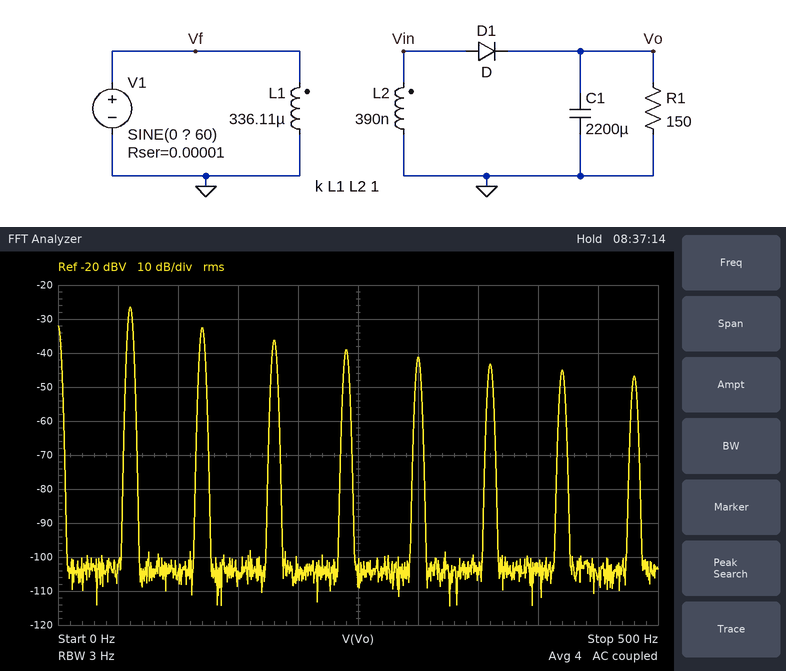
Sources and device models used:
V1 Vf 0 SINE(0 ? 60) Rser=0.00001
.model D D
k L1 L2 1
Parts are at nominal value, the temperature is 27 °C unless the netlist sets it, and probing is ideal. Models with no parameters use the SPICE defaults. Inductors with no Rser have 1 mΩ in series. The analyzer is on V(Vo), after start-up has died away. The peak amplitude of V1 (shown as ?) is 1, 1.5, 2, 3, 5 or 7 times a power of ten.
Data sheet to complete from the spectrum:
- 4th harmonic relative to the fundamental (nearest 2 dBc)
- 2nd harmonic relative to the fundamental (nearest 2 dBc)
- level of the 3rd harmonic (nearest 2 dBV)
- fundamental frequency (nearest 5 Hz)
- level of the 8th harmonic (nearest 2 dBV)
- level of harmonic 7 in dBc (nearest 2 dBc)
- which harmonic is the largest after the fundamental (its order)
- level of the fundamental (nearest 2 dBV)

-12 dBc
-6 dBc
-36 dBV
60 Hz
-46 dBV
-18 dBc
2
-26 dBV
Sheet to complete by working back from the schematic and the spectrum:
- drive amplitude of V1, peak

150 V
